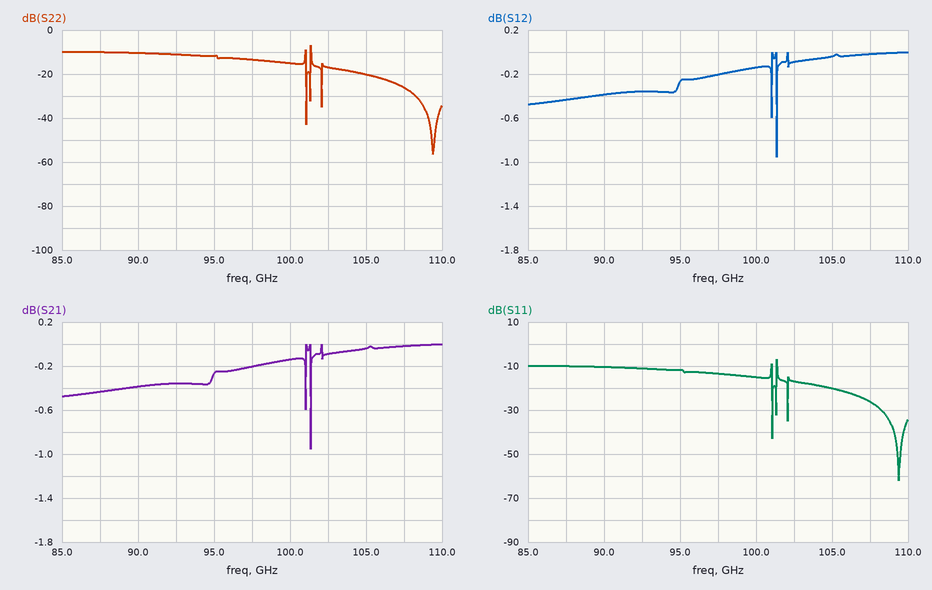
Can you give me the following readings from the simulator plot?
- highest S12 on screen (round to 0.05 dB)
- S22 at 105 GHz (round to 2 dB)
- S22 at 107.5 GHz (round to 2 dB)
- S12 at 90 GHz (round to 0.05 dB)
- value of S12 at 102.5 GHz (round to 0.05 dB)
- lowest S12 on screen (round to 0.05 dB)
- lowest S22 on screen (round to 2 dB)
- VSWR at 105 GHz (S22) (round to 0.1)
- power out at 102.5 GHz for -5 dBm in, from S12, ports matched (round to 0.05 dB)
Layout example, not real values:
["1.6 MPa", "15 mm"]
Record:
["0.00 dB", "-20 dB", "-26 dB", "-0.40 dB", "-0.10 dB", "-0.95 dB", "-56 dB", "1.2", "-5.10 dBm"]
